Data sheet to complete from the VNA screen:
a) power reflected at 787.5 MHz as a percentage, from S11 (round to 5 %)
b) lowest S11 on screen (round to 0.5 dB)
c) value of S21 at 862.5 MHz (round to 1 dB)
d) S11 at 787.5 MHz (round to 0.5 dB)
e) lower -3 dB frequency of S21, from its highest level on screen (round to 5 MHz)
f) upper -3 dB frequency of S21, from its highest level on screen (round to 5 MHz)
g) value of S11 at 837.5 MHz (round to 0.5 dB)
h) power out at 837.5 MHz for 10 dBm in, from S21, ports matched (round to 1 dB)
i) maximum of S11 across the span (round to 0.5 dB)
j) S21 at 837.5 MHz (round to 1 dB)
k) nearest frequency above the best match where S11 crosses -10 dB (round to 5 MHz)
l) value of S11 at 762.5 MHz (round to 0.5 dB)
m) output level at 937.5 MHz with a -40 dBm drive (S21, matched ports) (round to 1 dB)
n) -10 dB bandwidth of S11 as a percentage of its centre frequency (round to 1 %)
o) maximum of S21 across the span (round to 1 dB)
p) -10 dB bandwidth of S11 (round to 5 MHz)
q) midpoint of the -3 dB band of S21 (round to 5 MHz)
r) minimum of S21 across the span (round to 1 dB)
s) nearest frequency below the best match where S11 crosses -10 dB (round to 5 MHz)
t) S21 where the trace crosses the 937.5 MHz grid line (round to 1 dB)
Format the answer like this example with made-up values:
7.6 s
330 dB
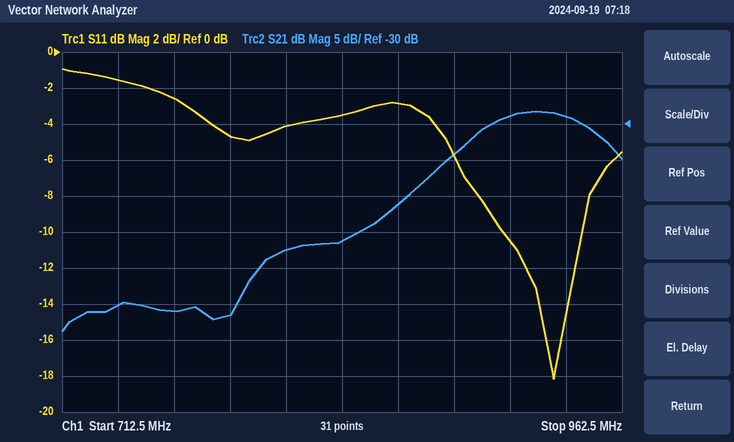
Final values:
35 %
-18.0 dB
-41 dB
-4.5 dB
900 MHz
950 MHz
-3.5 dB
-36 dBm
-1.0 dB
-46 dB
945 MHz
-2.5 dB
-69 dBm
4 %
-28 dB
35 MHz
925 MHz
-59 dB
910 MHz
-29 dB
